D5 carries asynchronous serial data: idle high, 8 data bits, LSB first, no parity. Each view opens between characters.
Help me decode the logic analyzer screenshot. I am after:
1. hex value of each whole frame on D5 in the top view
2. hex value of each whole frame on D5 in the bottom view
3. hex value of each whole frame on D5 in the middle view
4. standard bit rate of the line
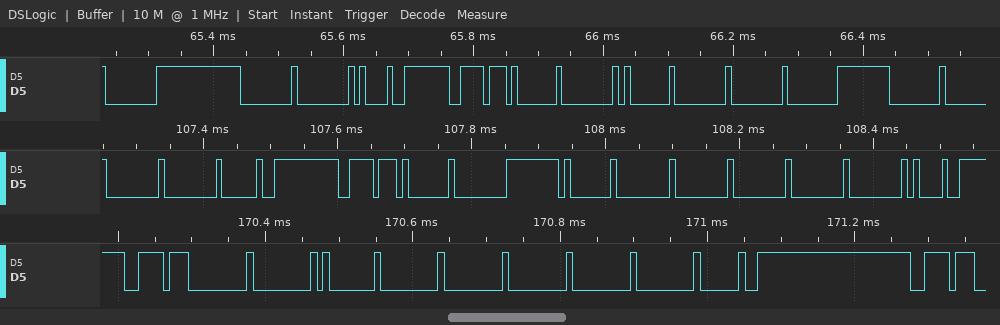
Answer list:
00, 00, 00, 21, DE, 01, 00, 01, 00, 00, 00, 00
DE, 00, 00, 01, 00, 00, 00, 00, 00, 20, DE
00, 00, 20, DE, 01, 00, 01, 00, 00, 00, 00, 00, 21
115200 baud
